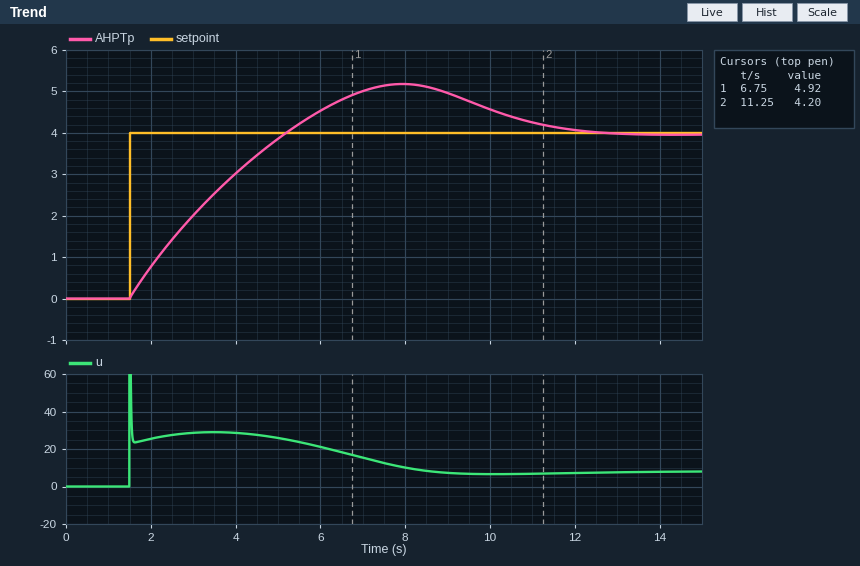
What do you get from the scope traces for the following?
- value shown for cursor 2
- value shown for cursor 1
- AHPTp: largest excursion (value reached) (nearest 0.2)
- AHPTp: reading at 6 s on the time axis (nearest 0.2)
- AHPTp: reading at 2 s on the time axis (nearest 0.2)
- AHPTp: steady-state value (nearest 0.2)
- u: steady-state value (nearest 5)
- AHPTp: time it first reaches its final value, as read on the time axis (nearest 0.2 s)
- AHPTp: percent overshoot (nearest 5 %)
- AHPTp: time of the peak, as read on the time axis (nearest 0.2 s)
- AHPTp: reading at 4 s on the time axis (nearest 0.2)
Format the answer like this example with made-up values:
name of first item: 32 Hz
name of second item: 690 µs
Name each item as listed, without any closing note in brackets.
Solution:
value shown for cursor 2: 4.20
value shown for cursor 1: 4.92
AHPTp: largest excursion (value reached): 5.2
AHPTp: reading at 6 s on the time axis: 4.6
AHPTp: reading at 2 s on the time axis: 0.8
AHPTp: steady-state value: 4.0
u: steady-state value: 10
AHPTp: time it first reaches its final value, as read on the time axis: 5.2 s
AHPTp: percent overshoot: 30 %
AHPTp: time of the peak, as read on the time axis: 8.0 s
AHPTp: reading at 4 s on the time axis: 3.0
